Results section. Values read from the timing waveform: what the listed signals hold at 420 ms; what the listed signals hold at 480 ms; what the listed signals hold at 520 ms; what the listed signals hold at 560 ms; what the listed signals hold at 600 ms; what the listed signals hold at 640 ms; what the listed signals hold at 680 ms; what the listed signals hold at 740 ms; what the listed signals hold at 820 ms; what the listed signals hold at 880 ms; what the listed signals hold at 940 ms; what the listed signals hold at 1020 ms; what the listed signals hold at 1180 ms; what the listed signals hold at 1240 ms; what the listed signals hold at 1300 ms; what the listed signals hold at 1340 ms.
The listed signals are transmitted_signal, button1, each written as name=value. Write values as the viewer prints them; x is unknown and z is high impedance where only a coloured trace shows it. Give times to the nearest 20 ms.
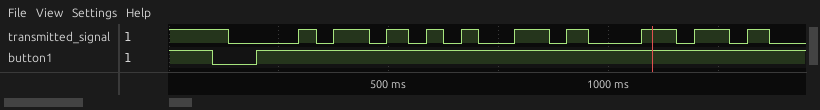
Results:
transmitted_signal=1, button1=1
transmitted_signal=0, button1=1
transmitted_signal=1, button1=1
transmitted_signal=0, button1=1
transmitted_signal=1, button1=1
transmitted_signal=0, button1=1
transmitted_signal=1, button1=1
transmitted_signal=0, button1=1
transmitted_signal=1, button1=1
transmitted_signal=0, button1=1
transmitted_signal=1, button1=1
transmitted_signal=0, button1=1
transmitted_signal=0, button1=1
transmitted_signal=1, button1=1
transmitted_signal=0, button1=1
transmitted_signal=1, button1=1
